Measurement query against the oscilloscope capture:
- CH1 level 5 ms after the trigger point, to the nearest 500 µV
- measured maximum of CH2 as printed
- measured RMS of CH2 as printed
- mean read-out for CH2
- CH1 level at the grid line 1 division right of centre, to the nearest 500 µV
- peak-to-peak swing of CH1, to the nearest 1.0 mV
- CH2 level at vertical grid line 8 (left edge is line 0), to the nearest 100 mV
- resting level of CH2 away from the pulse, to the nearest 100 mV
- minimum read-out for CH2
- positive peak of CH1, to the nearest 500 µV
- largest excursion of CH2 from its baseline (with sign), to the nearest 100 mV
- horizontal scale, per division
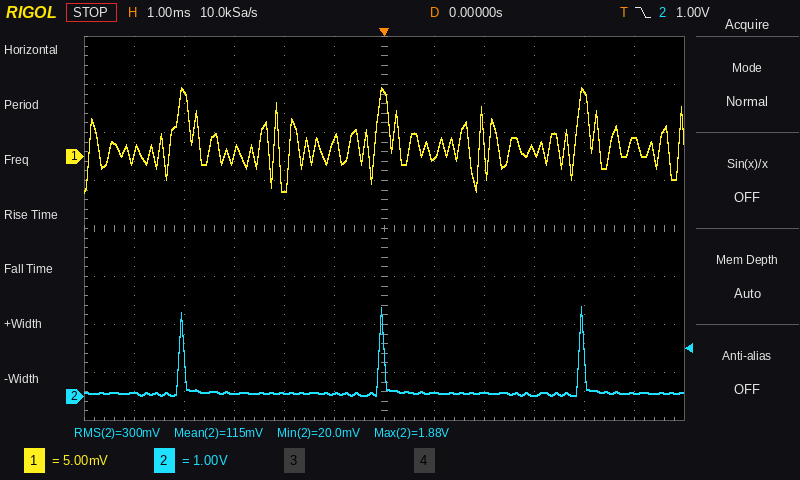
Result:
2.0 mV
1.88 V
300 mV
115 mV
0.0 mV
11.0 mV
100 mV
100 mV
20.0 mV
7.0 mV
+1.8 V
1 ms
